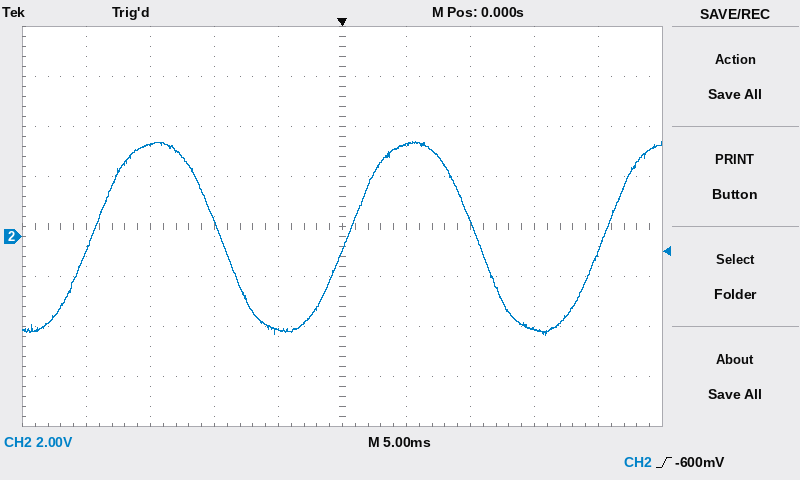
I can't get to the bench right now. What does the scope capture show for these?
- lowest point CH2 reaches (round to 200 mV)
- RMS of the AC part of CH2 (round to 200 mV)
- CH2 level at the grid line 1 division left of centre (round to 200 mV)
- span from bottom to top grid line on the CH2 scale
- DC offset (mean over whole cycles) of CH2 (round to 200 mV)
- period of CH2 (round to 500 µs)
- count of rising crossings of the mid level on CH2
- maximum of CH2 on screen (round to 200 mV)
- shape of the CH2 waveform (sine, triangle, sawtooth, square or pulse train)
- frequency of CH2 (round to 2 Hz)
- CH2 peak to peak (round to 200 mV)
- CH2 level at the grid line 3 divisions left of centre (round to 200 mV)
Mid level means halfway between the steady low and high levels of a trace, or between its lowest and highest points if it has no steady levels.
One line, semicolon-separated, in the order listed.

-4.0 V; 2.8 V; -3.8 V; 16 V; 0.0 V; 20.0 ms; 3; 3.8 V; sine; 50 Hz; 7.8 V; 3.6 V
